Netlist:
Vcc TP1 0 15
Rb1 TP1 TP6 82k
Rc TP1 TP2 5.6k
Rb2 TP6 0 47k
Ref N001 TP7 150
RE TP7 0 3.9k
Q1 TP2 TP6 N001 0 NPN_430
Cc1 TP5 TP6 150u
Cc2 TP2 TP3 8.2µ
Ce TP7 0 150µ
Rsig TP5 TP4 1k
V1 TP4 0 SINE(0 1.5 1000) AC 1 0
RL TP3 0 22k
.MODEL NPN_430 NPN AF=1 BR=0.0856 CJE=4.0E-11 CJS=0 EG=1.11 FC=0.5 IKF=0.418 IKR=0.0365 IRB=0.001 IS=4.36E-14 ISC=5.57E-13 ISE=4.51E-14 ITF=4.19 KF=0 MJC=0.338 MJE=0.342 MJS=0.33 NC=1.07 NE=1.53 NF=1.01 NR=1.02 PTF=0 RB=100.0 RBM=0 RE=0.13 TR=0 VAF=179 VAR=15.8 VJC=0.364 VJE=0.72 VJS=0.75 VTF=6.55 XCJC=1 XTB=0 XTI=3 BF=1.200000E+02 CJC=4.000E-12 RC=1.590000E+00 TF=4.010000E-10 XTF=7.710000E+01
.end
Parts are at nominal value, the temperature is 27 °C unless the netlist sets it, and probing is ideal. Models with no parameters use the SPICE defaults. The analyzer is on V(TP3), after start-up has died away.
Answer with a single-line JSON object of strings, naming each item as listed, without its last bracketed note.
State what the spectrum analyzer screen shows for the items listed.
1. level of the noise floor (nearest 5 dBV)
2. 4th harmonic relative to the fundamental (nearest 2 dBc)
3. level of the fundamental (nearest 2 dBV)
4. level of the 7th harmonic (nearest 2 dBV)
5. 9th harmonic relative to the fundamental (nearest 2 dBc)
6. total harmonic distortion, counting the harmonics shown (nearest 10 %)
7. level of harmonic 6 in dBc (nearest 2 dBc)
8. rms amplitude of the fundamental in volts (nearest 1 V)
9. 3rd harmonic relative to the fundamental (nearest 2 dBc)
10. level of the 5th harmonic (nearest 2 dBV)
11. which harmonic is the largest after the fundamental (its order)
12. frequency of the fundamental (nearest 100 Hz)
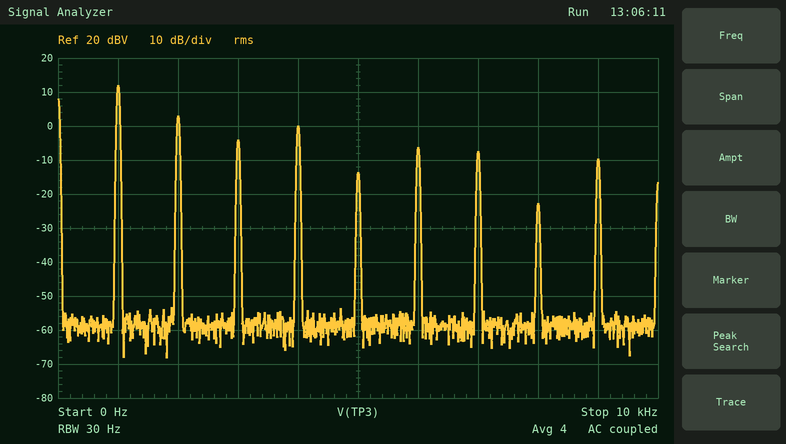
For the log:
{"level of the noise floor": "-60 dBV", "4th harmonic relative to the fundamental": "-12 dBc", "level of the fundamental": "12 dBV", "level of the 7th harmonic": "-8 dBV", "9th harmonic relative to the fundamental": "-22 dBc", "total harmonic distortion, counting the harmonics shown": "50 %", "level of harmonic 6 in dBc": "-18 dBc", "rms amplitude of the fundamental in volts": "4 V", "3rd harmonic relative to the fundamental": "-16 dBc", "level of the 5th harmonic": "-14 dBV", "which harmonic is the largest after the fundamental": "2", "frequency of the fundamental": "1.0 kHz"}
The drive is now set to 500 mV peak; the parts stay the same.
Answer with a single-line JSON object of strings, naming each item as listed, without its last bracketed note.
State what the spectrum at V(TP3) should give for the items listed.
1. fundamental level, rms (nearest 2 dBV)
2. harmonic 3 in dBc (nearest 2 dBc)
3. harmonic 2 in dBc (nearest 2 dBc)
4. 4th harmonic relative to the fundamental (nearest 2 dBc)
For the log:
{"fundamental level, rms": "12 dBV", "harmonic 3 in dBc": "-12 dBc", "harmonic 2 in dBc": "-22 dBc", "4th harmonic relative to the fundamental": "-26 dBc"}
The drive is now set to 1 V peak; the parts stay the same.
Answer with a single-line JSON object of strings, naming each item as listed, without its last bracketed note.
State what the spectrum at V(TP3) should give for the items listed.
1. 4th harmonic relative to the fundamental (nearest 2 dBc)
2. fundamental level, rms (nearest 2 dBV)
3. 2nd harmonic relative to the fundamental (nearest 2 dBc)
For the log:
{"4th harmonic relative to the fundamental": "-14 dBc", "fundamental level, rms": "12 dBV", "2nd harmonic relative to the fundamental": "-12 dBc"}
